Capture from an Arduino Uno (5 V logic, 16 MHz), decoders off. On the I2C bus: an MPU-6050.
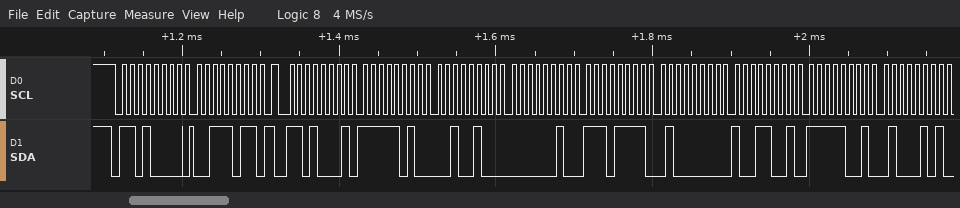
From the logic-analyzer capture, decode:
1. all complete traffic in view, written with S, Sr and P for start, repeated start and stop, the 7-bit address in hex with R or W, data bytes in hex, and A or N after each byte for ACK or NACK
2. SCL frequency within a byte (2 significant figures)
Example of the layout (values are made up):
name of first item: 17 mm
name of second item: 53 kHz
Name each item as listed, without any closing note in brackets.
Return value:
all complete traffic in view, written with S, Sr and P for start, repeated start and stop, the 7-bit address in hex with R or W, data bytes in hex, and A or N after each byte for ACK or NACK: S 68W A 3B A Sr 68R A FA A 24 A 02 A EF A 40 A 99 A F9 A 45 A
SCL frequency within a byte: 100 kHz
